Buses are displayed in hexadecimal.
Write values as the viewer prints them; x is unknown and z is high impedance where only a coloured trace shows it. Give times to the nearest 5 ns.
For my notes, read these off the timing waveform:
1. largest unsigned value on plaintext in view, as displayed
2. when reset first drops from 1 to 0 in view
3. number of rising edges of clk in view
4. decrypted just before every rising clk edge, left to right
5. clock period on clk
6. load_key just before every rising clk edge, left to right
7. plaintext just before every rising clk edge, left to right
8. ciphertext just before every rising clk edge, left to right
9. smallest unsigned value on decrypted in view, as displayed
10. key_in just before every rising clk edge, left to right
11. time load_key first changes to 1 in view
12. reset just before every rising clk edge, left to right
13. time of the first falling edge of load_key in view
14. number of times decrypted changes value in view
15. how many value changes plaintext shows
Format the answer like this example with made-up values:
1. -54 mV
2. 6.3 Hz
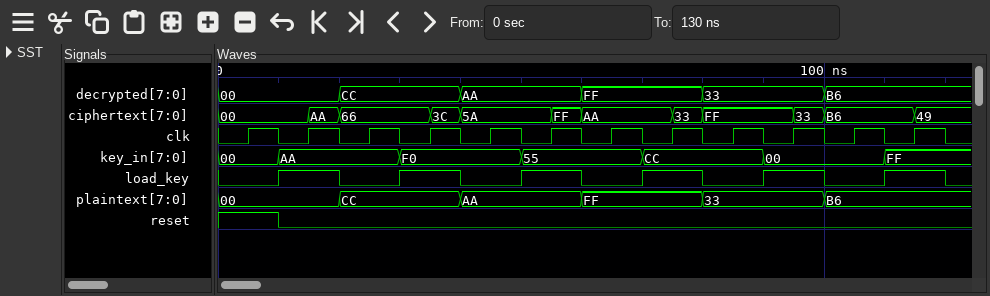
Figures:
1. FF
2. 10 ns
3. 12
4. 00, 00, CC, CC, AA, AA, FF, FF, 33, 33, B6, B6
5. 10 ns
6. 0 1 0 1 0 1 0 1 0 1 0 1
7. 00, 00, CC, CC, AA, AA, FF, FF, 33, 33, B6, B6
8. 00, 00, 66, 66, 5A, 5A, AA, AA, FF, FF, B6, B6
9. 00
10. 00, AA, AA, F0, F0, 55, 55, CC, CC, 00, 00, FF
11. 10 ns
12. 1 0 0 0 0 0 0 0 0 0 0 0
13. 20 ns
14. 5
15. 5
